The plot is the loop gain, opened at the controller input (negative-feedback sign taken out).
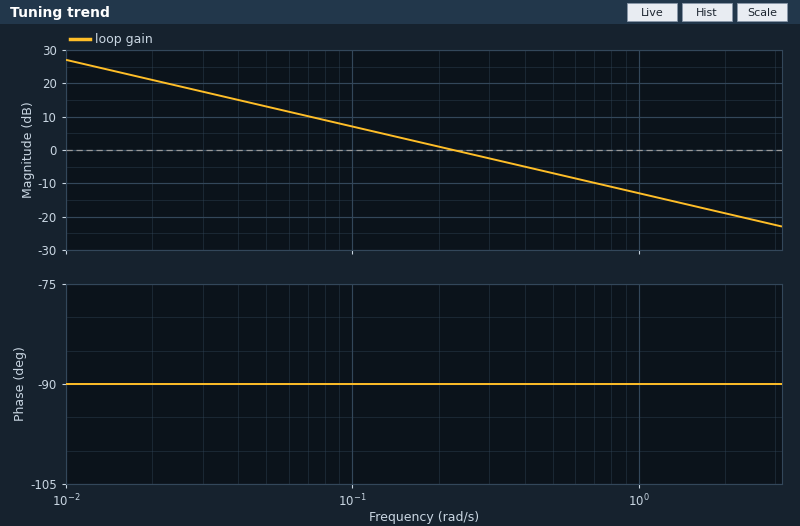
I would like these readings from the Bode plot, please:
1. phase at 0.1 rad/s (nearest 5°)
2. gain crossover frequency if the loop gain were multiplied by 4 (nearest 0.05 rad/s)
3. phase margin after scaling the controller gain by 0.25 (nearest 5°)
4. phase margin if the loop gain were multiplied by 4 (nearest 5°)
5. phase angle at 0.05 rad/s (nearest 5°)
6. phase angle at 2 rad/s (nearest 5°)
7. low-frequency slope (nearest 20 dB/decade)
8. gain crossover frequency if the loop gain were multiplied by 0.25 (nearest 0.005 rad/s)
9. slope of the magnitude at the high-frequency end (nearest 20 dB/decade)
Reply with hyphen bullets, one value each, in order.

- -90°
- 0.90 rad/s
- 90°
- 90°
- -90°
- -90°
- -20 dB/decade
- 0.055 rad/s
- -20 dB/decade
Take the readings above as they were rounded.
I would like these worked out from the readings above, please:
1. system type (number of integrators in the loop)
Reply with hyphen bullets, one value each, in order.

- 1
